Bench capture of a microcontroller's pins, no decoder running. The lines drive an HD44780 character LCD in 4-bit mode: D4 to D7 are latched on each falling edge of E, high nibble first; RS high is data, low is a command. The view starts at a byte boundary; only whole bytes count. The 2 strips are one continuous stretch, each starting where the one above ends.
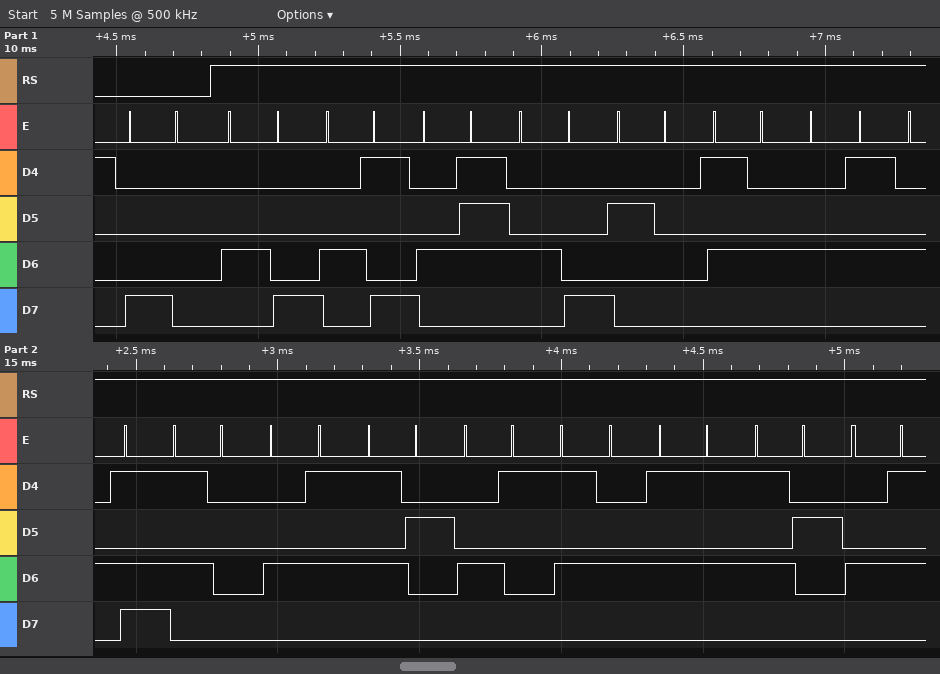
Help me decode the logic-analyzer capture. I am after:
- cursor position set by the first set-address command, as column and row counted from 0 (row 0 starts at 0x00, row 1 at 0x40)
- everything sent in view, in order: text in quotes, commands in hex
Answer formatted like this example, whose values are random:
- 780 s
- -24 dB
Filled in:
- column 0, row 0
- 0x80 "HIGH TEMPERATURE"
